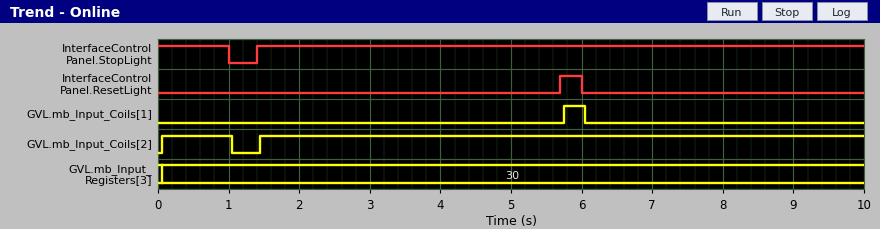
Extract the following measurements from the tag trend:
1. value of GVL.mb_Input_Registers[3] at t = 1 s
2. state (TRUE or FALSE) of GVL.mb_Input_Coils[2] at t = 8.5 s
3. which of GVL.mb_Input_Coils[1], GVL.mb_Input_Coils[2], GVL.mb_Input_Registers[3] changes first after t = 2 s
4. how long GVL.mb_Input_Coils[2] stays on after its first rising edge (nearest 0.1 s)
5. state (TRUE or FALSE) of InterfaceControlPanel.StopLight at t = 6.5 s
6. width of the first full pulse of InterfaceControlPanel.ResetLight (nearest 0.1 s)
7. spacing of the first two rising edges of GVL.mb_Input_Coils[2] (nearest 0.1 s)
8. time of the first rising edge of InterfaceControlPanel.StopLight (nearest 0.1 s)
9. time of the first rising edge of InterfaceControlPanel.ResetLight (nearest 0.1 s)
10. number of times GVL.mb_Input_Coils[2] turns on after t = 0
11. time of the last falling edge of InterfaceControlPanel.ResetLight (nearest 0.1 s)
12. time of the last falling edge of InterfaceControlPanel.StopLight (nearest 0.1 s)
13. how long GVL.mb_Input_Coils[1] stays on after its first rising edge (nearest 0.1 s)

30
TRUE
GVL.mb_Input_Coils[1]
1.0 s
TRUE
0.3 s
1.4 s
1.4 s
5.7 s
2
6.0 s
1.0 s
0.3 s
